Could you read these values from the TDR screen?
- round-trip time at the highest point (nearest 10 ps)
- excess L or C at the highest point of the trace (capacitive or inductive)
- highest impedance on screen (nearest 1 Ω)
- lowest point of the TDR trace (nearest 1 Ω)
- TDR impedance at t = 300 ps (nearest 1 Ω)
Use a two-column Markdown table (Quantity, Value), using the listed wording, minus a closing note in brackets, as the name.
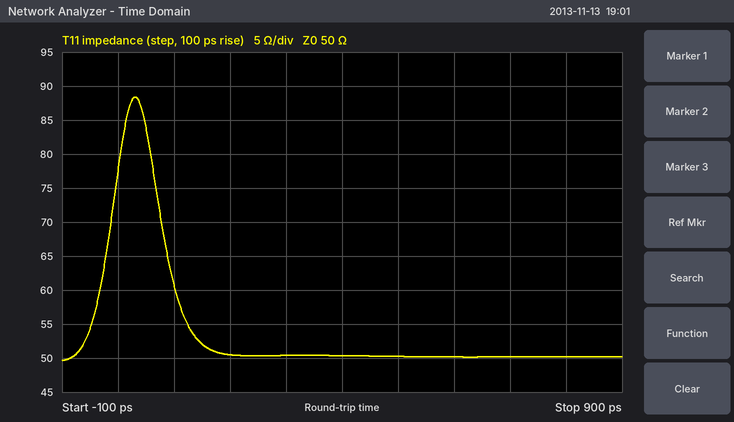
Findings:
| Quantity | Value |
|---|---|
| round-trip time at the highest point | 30 ps |
| excess L or C at the highest point of the trace | inductive |
| highest impedance on screen | 88 Ω |
| lowest point of the TDR trace | 50 Ω |
| TDR impedance at t = 300 ps | 50 Ω |
